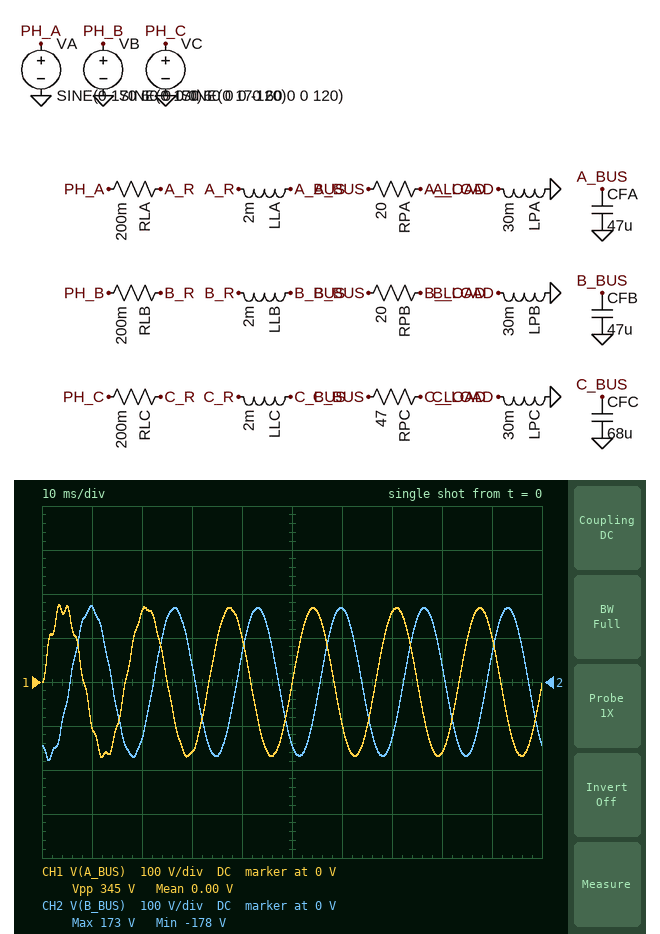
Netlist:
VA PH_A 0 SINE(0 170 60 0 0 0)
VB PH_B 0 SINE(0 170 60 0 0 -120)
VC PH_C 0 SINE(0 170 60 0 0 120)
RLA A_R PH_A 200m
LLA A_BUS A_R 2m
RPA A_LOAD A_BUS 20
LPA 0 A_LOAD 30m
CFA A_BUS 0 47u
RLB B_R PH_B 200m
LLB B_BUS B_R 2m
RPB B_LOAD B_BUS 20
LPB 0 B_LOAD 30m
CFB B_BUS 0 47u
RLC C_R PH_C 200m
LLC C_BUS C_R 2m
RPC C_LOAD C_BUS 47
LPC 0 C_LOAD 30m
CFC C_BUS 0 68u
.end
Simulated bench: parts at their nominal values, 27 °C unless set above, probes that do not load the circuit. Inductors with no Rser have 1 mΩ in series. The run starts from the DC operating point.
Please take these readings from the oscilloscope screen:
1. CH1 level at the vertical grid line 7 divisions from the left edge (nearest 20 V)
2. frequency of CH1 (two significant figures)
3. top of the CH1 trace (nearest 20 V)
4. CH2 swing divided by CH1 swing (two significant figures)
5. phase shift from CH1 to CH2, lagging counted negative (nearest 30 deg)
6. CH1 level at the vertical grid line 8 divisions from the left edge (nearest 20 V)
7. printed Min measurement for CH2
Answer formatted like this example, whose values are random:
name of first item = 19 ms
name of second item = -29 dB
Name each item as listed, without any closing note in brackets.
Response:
CH1 level at the vertical grid line 7 divisions from the left edge = 160 V
frequency of CH1 = 60 Hz
top of the CH1 trace = 180 V
CH2 swing divided by CH1 swing = 1.0
phase shift from CH1 to CH2, lagging counted negative = -120 deg
CH1 level at the vertical grid line 8 divisions from the left edge = -160 V
printed Min measurement for CH2 = -178 V
